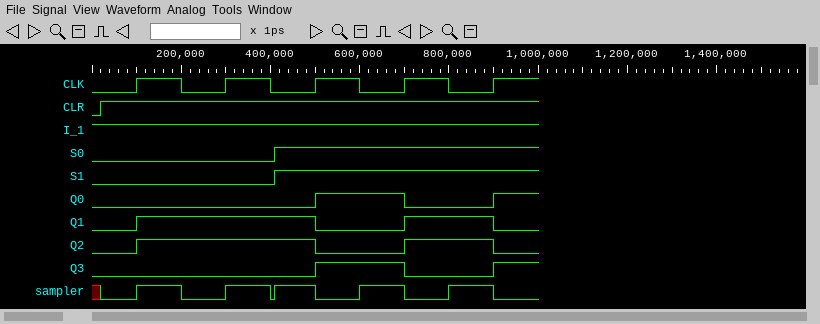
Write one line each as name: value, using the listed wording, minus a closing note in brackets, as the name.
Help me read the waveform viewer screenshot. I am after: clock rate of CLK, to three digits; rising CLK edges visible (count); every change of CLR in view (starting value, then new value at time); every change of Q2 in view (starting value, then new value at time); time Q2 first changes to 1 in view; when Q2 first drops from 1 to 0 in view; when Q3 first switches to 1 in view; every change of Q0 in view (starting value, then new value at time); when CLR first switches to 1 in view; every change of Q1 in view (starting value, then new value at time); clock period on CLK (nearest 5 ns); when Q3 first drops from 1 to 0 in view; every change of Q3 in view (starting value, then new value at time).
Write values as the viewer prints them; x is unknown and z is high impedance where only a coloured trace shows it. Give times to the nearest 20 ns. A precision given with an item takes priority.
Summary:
clock rate of CLK, to three digits: 5.00 MHz
rising CLK edges visible: 5
every change of CLR in view: 0, 1 at 20 ns
every change of Q2 in view: 0, 1 at 100 ns, 0 at 500 ns, 1 at 700 ns, 0 at 900 ns
time Q2 first changes to 1 in view: 100 ns
when Q2 first drops from 1 to 0 in view: 500 ns
when Q3 first switches to 1 in view: 500 ns
every change of Q0 in view: 0, 1 at 500 ns, 0 at 700 ns, 1 at 900 ns
when CLR first switches to 1 in view: 20 ns
every change of Q1 in view: 0, 1 at 100 ns, 0 at 500 ns, 1 at 700 ns, 0 at 900 ns
clock period on CLK: 200 ns
when Q3 first drops from 1 to 0 in view: 700 ns
every change of Q3 in view: 0, 1 at 500 ns, 0 at 700 ns, 1 at 900 ns
